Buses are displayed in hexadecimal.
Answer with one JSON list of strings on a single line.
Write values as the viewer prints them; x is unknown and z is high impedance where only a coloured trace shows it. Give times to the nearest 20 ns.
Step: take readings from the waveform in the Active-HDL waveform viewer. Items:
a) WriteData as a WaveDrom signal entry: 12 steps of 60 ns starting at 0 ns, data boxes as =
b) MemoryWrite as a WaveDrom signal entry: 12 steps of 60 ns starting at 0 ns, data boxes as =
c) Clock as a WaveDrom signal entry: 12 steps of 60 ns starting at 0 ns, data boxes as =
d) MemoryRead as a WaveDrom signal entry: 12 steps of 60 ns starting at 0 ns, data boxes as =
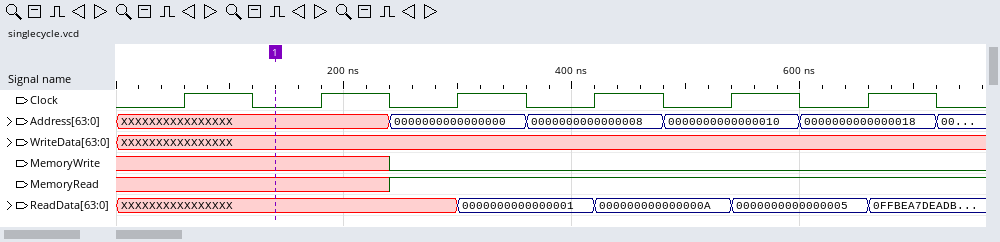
["{name: 'WriteData', wave: 'x...........'}", "{name: 'MemoryWrite', wave: 'x...0.......'}", "{name: 'Clock', wave: '010101010101'}", "{name: 'MemoryRead', wave: 'x...1.......'}"]
